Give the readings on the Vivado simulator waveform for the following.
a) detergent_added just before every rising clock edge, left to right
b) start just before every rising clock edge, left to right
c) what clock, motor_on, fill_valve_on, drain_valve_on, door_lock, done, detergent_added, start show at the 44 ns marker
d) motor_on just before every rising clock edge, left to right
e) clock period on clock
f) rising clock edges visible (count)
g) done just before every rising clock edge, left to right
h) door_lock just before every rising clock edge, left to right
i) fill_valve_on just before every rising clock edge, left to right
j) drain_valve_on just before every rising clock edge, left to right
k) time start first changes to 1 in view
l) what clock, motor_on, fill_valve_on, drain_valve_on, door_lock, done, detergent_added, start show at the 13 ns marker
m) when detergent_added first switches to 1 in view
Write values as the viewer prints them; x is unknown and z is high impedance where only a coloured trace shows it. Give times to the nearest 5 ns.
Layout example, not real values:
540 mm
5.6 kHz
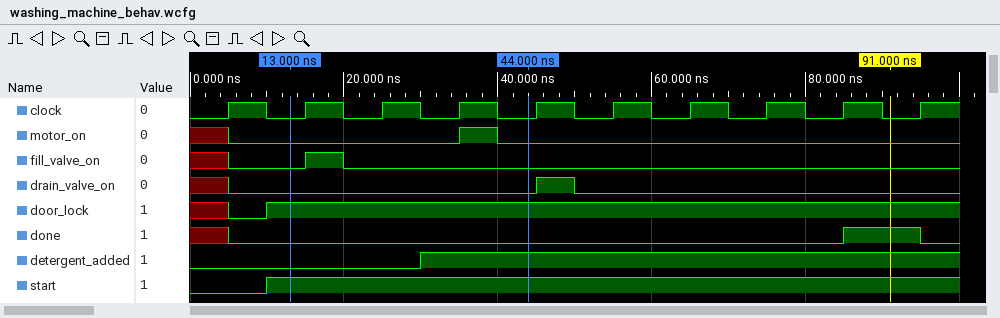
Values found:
0 0 0 1 1 1 1 1 1 1
0 1 1 1 1 1 1 1 1 1
clock=0, motor_on=0, fill_valve_on=0, drain_valve_on=0, door_lock=1, done=0, detergent_added=1, start=1
x 0 0 0 0 0 0 0 0 0
10 ns
10
x 0 0 0 0 0 0 0 0 1
x 1 1 1 1 1 1 1 1 1
x 0 0 0 0 0 0 0 0 0
x 0 0 0 0 0 0 0 0 0
10 ns
clock=0, motor_on=0, fill_valve_on=0, drain_valve_on=0, door_lock=1, done=0, detergent_added=0, start=1
30 ns
